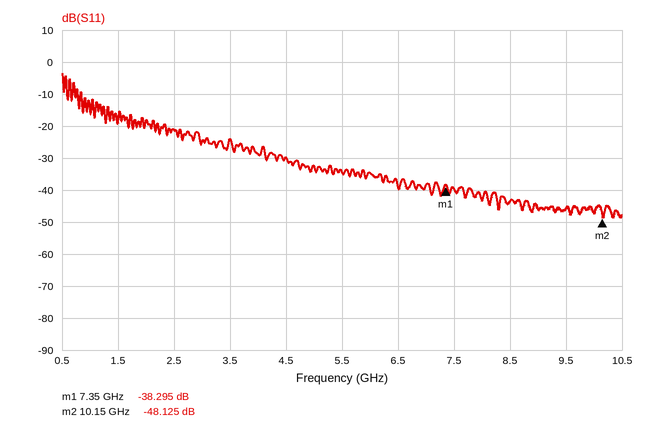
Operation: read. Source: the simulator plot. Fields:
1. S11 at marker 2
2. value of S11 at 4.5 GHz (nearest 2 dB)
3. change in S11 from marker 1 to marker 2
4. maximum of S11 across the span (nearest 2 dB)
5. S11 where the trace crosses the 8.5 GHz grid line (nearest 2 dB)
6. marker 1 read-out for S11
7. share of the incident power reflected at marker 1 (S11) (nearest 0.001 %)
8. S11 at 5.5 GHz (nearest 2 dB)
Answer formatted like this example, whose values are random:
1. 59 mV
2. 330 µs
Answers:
1. -48.125 dB
2. -30 dB
3. -9.830 dB
4. -4 dB
5. -44 dB
6. -38.295 dB
7. 0.015 %
8. -34 dB
